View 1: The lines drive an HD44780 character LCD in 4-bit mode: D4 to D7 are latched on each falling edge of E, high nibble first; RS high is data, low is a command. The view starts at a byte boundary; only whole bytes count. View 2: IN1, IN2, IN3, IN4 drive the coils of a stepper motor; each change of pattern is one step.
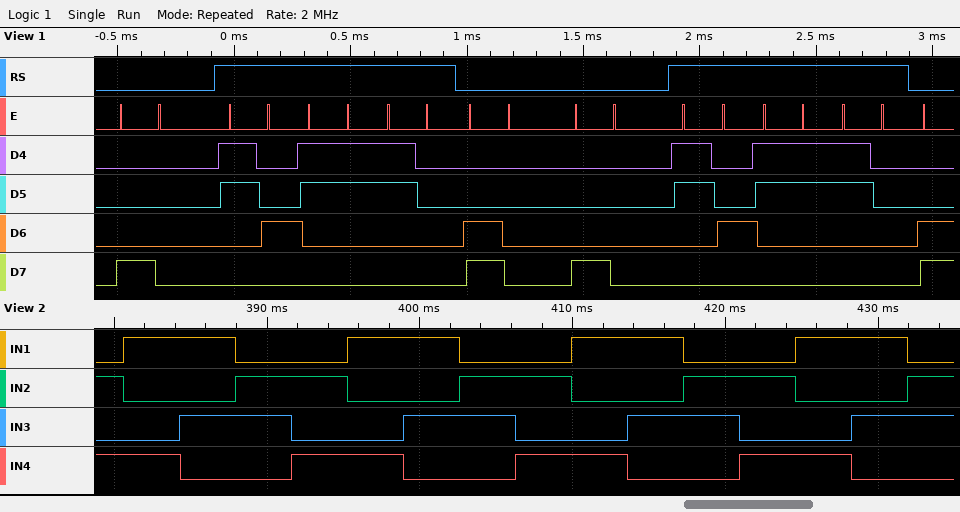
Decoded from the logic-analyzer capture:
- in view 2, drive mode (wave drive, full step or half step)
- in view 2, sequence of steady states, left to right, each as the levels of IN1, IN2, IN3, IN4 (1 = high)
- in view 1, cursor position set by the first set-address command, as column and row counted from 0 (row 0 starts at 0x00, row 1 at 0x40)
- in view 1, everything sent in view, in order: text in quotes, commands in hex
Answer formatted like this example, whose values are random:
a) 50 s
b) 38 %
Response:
a) full step
b) 0101 1001 1010 0110 0101 1001 1010 0110 0101 1001 1010 0110 0101 1001 1010 0110
c) column 0, row 0
d) 0x80 "430" 0xC0 0x80 "430"
